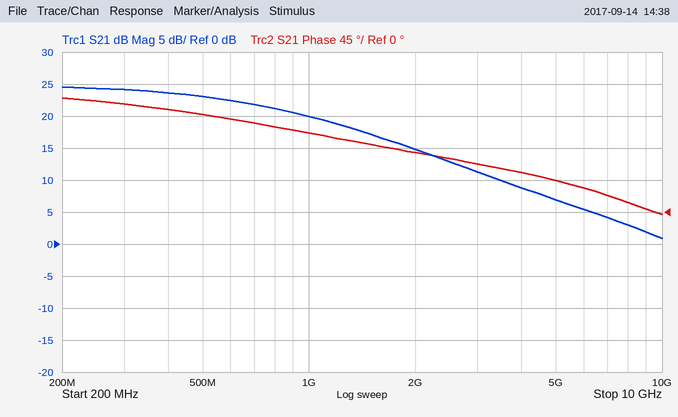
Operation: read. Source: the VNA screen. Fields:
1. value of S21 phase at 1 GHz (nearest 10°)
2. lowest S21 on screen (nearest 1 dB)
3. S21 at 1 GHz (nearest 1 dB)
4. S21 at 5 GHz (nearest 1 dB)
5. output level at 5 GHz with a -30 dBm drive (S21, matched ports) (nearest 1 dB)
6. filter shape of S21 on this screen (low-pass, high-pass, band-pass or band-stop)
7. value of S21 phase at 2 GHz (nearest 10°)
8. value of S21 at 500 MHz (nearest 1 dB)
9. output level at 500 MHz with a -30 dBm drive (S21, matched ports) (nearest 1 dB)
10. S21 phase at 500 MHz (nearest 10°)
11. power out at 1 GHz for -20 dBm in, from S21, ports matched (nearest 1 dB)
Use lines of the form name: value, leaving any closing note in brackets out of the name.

value of S21 phase at 1 GHz: 110°
lowest S21 on screen: 1 dB
S21 at 1 GHz: 20 dB
S21 at 5 GHz: 7 dB
output level at 5 GHz with a -30 dBm drive (S21, matched ports): -23 dBm
filter shape of S21 on this screen: low-pass
value of S21 phase at 2 GHz: 80°
value of S21 at 500 MHz: 23 dB
output level at 500 MHz with a -30 dBm drive (S21, matched ports): -7 dBm
S21 phase at 500 MHz: 140°
power out at 1 GHz for -20 dBm in, from S21, ports matched: 0 dBm
